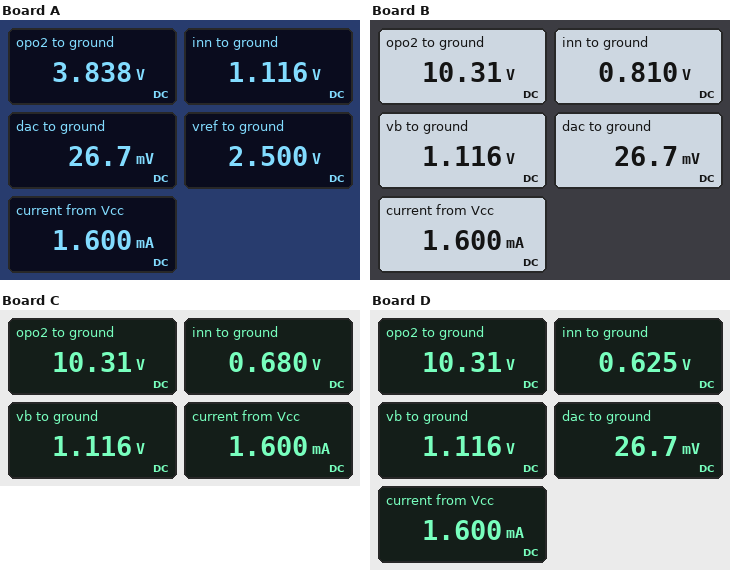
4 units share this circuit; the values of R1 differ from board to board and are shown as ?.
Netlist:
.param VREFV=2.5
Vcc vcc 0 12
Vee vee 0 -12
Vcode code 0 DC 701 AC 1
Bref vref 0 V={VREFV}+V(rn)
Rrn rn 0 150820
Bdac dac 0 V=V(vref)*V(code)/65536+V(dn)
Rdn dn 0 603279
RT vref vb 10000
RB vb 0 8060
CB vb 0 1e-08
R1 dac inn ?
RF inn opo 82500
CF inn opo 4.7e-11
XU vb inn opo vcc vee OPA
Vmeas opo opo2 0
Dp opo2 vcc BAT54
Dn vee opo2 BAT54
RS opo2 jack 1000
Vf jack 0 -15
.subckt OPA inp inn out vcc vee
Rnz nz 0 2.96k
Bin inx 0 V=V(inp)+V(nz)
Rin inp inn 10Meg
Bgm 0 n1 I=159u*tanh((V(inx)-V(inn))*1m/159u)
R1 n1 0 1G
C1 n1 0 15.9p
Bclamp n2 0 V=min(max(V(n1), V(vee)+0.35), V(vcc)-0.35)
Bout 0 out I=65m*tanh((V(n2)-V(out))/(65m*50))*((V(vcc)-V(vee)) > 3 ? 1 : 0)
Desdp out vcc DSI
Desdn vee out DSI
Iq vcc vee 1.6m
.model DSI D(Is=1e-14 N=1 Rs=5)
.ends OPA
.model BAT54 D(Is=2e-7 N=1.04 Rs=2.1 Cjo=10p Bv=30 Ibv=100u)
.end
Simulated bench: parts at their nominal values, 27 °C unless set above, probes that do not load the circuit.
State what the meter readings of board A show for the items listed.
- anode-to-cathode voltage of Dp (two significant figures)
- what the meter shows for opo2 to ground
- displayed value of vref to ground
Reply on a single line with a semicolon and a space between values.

-8.2 V; 3.838 V; 2.500 V
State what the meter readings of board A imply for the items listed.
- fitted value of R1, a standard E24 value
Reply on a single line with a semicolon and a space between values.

33 kΩ
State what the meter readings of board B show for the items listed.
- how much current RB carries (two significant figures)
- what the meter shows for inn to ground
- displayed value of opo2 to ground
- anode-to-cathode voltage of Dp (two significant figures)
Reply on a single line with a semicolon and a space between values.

140 µA; 0.810 V; 10.31 V; -1.7 V
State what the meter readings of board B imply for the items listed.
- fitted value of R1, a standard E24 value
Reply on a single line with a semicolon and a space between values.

6.8 kΩ
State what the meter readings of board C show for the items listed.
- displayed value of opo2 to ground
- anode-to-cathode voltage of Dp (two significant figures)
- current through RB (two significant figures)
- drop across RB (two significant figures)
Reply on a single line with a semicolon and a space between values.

10.31 V; -1.7 V; 140 µA; 1.1 V
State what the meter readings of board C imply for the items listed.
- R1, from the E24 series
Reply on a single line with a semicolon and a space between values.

5.6 kΩ
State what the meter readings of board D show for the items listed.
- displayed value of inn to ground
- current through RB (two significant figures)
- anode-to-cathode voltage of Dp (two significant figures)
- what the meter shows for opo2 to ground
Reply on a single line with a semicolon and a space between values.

0.625 V; 140 µA; -1.7 V; 10.31 V
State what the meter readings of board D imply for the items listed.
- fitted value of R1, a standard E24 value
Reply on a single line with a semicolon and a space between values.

5.1 kΩ
